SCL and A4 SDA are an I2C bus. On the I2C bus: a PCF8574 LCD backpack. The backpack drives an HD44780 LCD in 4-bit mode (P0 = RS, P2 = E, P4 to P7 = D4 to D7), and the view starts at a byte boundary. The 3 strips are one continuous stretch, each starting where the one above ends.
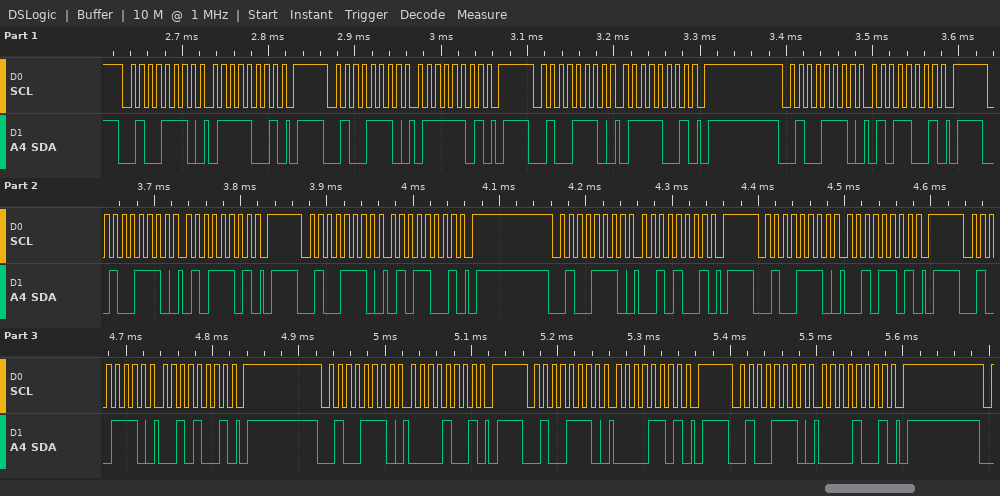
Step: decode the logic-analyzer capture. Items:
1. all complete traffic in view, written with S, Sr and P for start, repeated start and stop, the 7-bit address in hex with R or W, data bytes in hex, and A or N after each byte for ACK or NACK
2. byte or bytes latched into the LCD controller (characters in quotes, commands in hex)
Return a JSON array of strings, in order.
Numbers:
["S 27W A 79 A P S 27W A 7D A P S 27W A 79 A P S 27W A 59 A P S 27W A 5D A P S 27W A 59 A P S 27W A 29 A P S 27W A 2D A P S 27W A 29 A P S 27W A 09 A P S 27W A 0D A P S 27W A 09 A P", "'u' ' '"]
